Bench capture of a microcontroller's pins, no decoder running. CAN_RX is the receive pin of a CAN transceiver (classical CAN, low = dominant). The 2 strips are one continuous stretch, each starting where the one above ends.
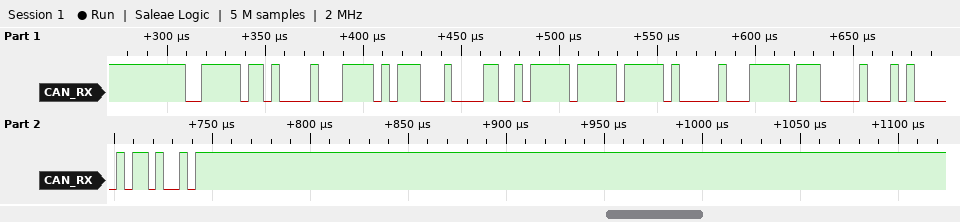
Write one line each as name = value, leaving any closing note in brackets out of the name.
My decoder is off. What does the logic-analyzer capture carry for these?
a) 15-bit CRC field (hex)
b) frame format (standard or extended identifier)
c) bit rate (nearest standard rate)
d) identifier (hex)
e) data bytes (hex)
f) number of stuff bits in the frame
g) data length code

15-bit CRC field = 0x5034
frame format = standard
bit rate = 250 kbit/s
identifier = 0x3FA
data bytes = F5 C4 32 FF FF 00 FF 00
number of stuff bits in the frame = 8
data length code = 8
